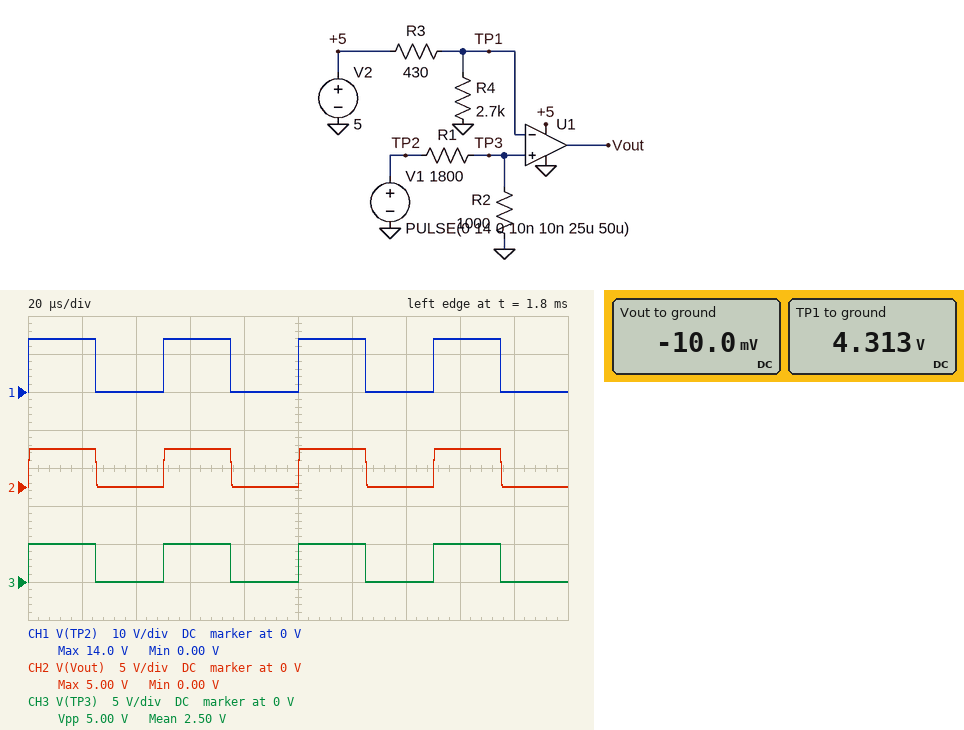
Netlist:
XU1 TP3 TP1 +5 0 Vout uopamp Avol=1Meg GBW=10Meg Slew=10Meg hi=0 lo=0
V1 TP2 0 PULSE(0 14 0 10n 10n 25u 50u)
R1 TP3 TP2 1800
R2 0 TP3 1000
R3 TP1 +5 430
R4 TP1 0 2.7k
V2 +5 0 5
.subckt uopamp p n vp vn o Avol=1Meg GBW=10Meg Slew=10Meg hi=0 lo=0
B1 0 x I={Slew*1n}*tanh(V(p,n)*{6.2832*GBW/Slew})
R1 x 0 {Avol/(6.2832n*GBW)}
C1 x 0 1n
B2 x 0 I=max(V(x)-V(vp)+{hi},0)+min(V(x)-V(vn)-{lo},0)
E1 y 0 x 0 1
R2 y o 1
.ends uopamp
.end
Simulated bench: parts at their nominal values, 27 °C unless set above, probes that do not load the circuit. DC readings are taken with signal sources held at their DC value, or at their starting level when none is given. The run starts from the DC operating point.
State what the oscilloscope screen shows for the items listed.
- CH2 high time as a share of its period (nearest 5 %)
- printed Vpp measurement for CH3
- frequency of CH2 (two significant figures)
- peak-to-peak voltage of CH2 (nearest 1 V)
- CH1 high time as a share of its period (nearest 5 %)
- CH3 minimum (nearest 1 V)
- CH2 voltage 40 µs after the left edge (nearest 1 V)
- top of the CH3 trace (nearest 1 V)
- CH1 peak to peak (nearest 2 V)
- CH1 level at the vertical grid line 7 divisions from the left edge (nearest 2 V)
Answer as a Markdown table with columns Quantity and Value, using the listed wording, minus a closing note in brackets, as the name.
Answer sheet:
| Quantity | Value |
|---|---|
| CH2 high time as a share of its period | 50 % |
| printed Vpp measurement for CH3 | 5.00 V |
| frequency of CH2 | 20 kHz |
| peak-to-peak voltage of CH2 | 5 V |
| CH1 high time as a share of its period | 50 % |
| CH3 minimum | 0 V |
| CH2 voltage 40 µs after the left edge | 0 V |
| top of the CH3 trace | 5 V |
| CH1 peak to peak | 14 V |
| CH1 level at the vertical grid line 7 divisions from the left edge | 0 V |
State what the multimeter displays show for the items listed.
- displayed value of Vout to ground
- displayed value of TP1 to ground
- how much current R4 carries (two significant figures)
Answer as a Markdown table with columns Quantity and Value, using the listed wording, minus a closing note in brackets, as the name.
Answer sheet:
| Quantity | Value |
|---|---|
| displayed value of Vout to ground | -10.0 mV |
| displayed value of TP1 to ground | 4.313 V |
| how much current R4 carries | 1.6 mA |
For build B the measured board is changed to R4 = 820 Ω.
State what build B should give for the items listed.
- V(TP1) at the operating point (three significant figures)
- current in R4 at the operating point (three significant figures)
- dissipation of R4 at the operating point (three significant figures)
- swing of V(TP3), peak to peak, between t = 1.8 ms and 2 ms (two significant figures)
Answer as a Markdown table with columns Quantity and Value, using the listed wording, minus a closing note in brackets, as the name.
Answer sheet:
| Quantity | Value |
|---|---|
| V(TP1) at the operating point | 3.28 V |
| current in R4 at the operating point | 4.00 mA |
| dissipation of R4 at the operating point | 13.1 mW |
| swing of V(TP3), peak to peak, between t = 1.8 ms and 2 ms | 5.0 V |
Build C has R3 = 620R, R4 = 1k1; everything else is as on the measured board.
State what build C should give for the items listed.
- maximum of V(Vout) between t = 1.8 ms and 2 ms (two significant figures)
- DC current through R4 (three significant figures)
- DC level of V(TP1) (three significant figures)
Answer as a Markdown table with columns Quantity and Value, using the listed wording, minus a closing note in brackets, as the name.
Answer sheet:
| Quantity | Value |
|---|---|
| maximum of V(Vout) between t = 1.8 ms and 2 ms | 5.0 V |
| DC current through R4 | 2.91 mA |
| DC level of V(TP1) | 3.20 V |
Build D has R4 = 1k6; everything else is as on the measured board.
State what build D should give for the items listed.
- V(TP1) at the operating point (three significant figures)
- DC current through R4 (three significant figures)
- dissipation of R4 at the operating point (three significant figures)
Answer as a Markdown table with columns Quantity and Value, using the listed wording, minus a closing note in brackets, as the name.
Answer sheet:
| Quantity | Value |
|---|---|
| V(TP1) at the operating point | 3.94 V |
| DC current through R4 | 2.46 mA |
| dissipation of R4 at the operating point | 9.71 mW |
